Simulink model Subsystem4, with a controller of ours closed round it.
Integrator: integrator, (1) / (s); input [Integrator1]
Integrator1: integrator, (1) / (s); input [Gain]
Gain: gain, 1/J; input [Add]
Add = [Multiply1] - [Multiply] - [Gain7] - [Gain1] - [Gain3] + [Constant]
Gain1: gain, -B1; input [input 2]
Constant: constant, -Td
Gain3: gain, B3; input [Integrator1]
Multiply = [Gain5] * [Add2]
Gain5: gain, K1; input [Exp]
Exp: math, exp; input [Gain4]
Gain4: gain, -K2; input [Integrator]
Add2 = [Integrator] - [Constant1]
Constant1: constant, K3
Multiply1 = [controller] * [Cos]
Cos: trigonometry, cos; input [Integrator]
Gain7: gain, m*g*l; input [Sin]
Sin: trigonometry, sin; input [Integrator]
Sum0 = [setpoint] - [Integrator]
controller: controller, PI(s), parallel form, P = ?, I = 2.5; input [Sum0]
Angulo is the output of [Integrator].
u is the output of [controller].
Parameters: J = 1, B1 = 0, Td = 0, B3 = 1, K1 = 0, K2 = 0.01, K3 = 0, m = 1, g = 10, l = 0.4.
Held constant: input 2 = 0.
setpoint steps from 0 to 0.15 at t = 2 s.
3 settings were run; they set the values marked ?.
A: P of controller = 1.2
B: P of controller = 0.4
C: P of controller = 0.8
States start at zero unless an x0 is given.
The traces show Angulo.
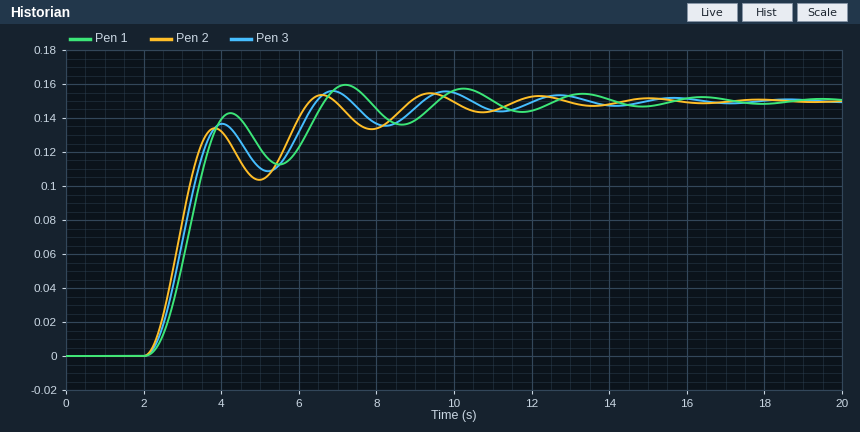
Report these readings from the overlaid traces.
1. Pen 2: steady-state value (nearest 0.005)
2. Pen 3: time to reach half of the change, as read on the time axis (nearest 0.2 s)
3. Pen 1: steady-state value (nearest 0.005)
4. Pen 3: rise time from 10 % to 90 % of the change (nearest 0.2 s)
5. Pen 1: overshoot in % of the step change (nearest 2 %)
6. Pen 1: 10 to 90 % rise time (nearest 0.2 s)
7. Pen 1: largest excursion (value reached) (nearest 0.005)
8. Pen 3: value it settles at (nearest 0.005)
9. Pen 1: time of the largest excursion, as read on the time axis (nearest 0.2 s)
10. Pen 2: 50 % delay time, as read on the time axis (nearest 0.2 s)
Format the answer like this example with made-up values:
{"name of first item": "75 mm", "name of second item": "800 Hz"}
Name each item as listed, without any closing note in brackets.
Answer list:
{"Pen 2: steady-state value": "0.150", "Pen 3: time to reach half of the change, as read on the time axis": "3.0 s", "Pen 1: steady-state value": "0.150", "Pen 3: rise time from 10 % to 90 % of the change": "1.4 s", "Pen 1: overshoot in % of the step change": "6 %", "Pen 1: 10 to 90 % rise time": "1.4 s", "Pen 1: largest excursion (value reached)": "0.160", "Pen 3: value it settles at": "0.150", "Pen 1: time of the largest excursion, as read on the time axis": "7.2 s", "Pen 2: 50 % delay time, as read on the time axis": "3.0 s"}
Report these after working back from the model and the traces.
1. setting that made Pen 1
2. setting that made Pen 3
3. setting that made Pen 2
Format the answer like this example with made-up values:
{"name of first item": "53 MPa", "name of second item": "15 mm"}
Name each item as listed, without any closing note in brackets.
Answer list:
{"setting that made Pen 1": "B", "setting that made Pen 3": "C", "setting that made Pen 2": "A"}
